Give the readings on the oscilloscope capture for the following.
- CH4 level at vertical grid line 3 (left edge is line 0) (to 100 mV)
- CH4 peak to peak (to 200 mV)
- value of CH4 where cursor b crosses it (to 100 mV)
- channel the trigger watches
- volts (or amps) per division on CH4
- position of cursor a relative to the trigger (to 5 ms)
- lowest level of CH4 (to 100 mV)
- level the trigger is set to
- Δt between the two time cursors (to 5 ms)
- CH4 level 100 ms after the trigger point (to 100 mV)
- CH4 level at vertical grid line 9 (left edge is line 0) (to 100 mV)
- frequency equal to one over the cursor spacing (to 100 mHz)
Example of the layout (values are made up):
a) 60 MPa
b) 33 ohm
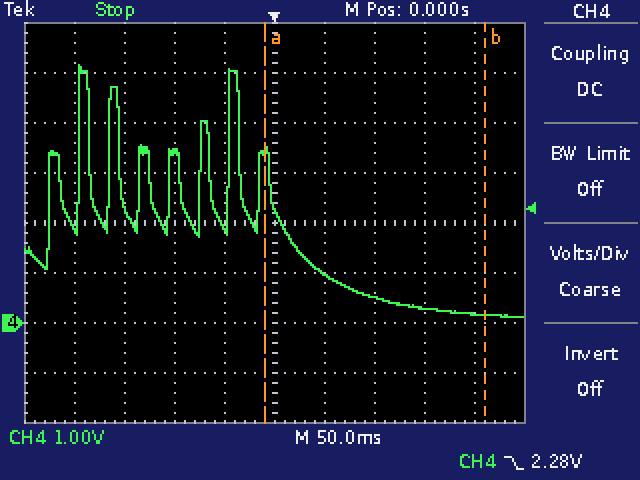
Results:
a) 3.4 V
b) 5.0 V
c) 200 mV
d) CH4
e) 1 V
f) -10 ms
g) 100 mV
h) 2.28 V
i) 220 ms
j) 500 mV
k) 200 mV
l) 4.5 Hz
